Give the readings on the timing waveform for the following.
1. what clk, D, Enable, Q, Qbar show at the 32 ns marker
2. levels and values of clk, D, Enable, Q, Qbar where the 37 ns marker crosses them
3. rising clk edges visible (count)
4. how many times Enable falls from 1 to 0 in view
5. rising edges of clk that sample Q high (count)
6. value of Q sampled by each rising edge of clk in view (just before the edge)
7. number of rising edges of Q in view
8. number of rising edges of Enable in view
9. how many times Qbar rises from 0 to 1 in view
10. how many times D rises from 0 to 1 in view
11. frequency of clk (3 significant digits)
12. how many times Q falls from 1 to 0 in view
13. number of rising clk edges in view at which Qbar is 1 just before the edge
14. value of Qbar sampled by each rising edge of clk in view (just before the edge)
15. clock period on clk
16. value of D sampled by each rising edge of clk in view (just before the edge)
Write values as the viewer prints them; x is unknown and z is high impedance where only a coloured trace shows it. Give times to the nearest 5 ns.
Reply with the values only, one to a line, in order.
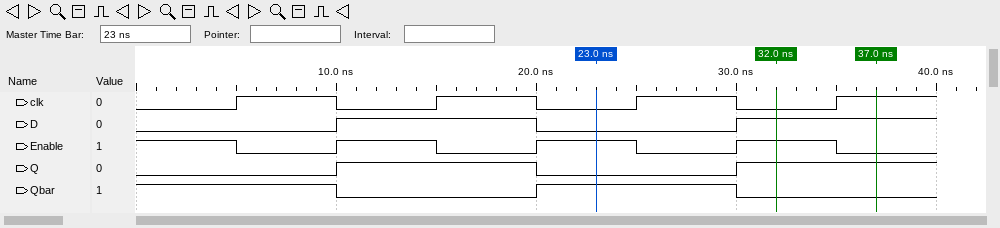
clk=0, D=1, Enable=1, Q=1, Qbar=0
clk=1, D=1, Enable=0, Q=1, Qbar=0
4
4
2
0 1 0 1
2
3
1
2
100 MHz
1
2
1 0 1 0
10 ns
0 1 0 1
